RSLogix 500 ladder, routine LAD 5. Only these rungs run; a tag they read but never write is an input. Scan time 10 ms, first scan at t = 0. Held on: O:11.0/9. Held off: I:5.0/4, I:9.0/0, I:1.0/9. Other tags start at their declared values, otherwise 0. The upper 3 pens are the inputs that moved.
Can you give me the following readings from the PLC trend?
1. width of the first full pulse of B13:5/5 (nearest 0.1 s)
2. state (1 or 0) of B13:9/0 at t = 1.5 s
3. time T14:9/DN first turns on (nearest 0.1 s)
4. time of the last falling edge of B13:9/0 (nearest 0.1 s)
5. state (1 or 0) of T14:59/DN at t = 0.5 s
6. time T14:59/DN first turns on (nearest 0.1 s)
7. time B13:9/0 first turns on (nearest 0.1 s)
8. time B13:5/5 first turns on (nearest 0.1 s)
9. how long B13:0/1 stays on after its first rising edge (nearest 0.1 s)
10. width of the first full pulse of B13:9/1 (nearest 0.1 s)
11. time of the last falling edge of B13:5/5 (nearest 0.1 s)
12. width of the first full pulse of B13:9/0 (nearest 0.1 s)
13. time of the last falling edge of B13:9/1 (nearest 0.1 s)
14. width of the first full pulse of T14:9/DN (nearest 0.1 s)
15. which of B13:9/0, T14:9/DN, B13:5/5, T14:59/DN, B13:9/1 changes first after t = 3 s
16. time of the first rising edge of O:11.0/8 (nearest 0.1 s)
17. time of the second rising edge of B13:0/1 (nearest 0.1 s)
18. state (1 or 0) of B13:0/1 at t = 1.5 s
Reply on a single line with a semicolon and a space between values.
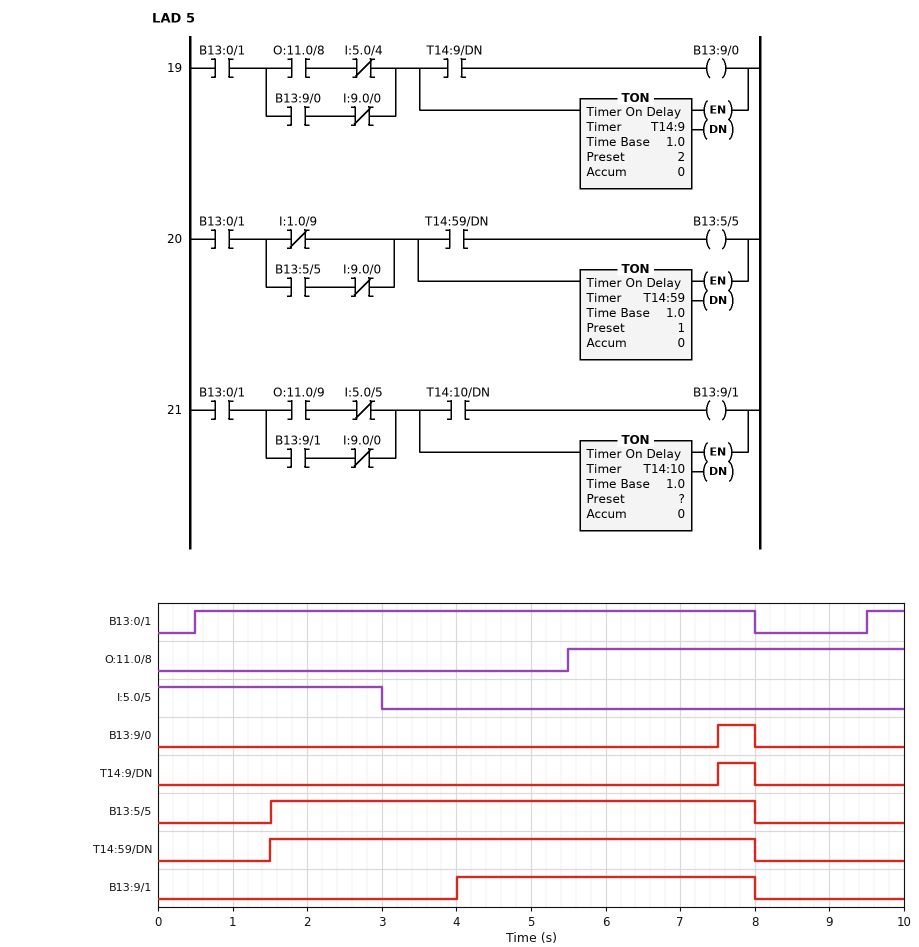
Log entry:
6.5 s; 0; 7.5 s; 8.0 s; 0; 1.5 s; 7.5 s; 1.5 s; 7.5 s; 4.0 s; 8.0 s; 0.5 s; 8.0 s; 0.5 s; B13:9/1; 5.5 s; 9.5 s; 1
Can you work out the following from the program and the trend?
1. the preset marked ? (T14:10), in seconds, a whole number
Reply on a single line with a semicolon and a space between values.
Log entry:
1 s
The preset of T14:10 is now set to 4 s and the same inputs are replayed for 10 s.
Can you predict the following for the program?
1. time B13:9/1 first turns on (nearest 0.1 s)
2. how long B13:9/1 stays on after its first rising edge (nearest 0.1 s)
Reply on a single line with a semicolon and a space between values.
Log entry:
7.0 s; 1.0 s
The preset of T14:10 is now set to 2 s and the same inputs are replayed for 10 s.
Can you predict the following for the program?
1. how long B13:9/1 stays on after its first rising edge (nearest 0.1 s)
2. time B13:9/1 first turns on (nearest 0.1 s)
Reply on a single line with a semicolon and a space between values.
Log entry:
3.0 s; 5.0 s
